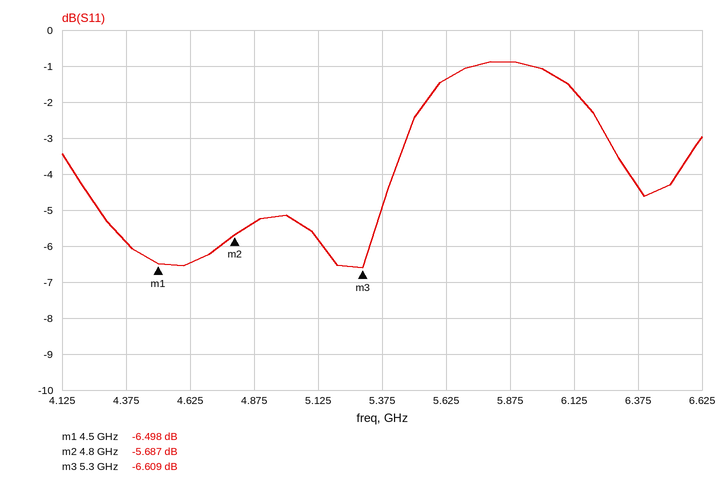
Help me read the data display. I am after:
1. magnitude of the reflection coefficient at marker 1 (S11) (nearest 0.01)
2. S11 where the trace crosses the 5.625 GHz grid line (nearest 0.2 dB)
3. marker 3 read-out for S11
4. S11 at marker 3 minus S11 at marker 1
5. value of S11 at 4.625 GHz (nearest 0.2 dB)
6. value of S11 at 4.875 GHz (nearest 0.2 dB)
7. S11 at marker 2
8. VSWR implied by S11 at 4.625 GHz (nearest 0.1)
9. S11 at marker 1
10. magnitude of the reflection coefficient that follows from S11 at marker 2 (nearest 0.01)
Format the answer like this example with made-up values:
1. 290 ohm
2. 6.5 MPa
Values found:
1. 0.47
2. -1.4 dB
3. -6.609 dB
4. -0.111 dB
5. -6.4 dB
6. -5.4 dB
7. -5.687 dB
8. 2.8
9. -6.498 dB
10. 0.52
